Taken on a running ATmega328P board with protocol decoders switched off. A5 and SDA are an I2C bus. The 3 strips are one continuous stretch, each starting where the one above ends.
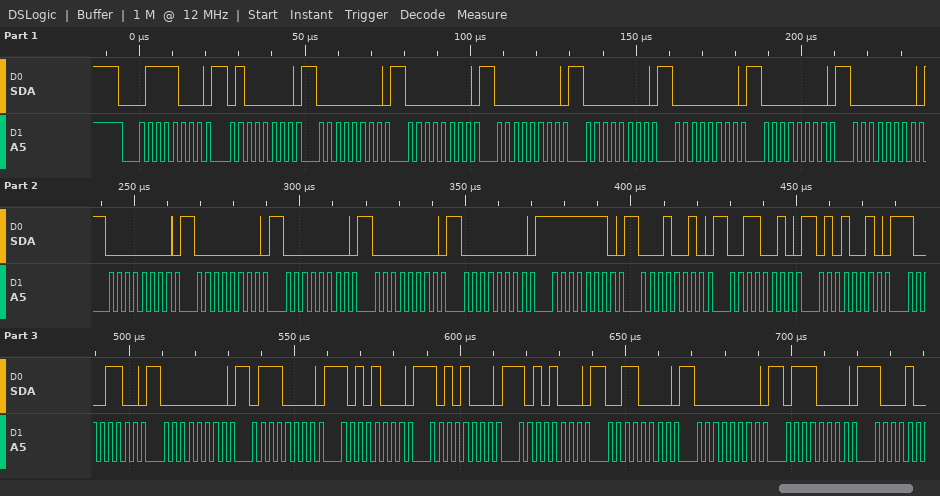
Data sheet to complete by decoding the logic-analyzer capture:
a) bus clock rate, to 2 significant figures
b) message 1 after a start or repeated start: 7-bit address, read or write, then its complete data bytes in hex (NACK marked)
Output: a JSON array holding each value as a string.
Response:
["400 kHz", "0x3C write: 40 00 00 00 00 00 00 00 00 00 00 00 00 FE 12 32 52 8C 00 70 A8 A8 A8 30 00 70"]
